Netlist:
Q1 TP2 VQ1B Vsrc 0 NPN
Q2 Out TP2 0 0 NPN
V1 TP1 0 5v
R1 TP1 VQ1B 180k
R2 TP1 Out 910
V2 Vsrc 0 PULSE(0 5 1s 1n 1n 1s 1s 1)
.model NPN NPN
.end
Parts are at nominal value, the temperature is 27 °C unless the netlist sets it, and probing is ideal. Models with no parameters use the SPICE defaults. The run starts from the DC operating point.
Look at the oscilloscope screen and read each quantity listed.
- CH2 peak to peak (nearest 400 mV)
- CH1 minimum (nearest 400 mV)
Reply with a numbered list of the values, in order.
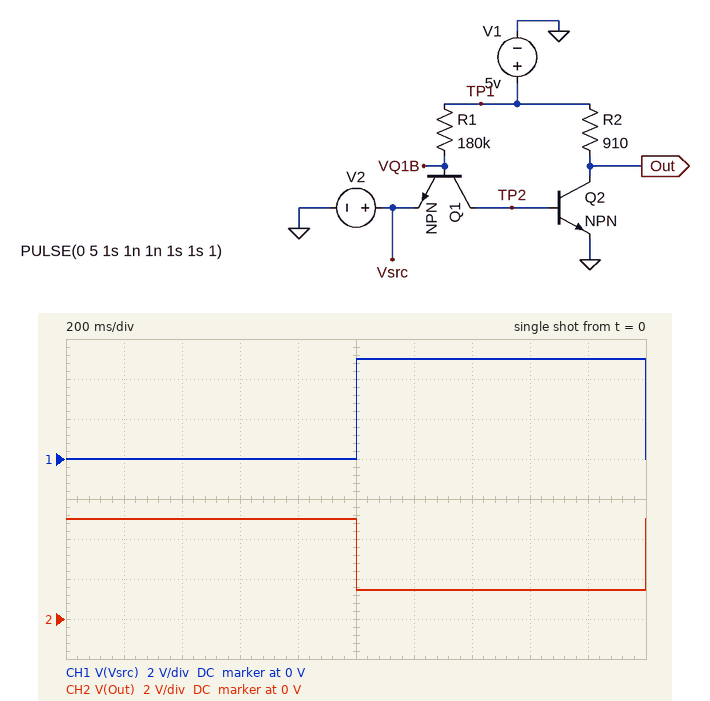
1. 3.6 V
2. 0 V
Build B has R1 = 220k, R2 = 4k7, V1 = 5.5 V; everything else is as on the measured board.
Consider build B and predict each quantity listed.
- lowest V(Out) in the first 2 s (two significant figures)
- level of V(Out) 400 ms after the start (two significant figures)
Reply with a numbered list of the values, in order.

1. 100 mV
2. 5.5 V
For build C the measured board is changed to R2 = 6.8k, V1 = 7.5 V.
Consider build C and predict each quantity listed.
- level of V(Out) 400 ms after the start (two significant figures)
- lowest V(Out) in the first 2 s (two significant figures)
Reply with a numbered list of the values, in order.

1. 7.5 V
2. 80 mV
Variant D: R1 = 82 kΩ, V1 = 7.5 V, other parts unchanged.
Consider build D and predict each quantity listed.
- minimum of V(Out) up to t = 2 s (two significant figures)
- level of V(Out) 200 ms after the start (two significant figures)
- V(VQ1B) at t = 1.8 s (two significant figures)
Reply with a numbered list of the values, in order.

1. 130 mV
2. 7.5 V
3. 1.5 V
